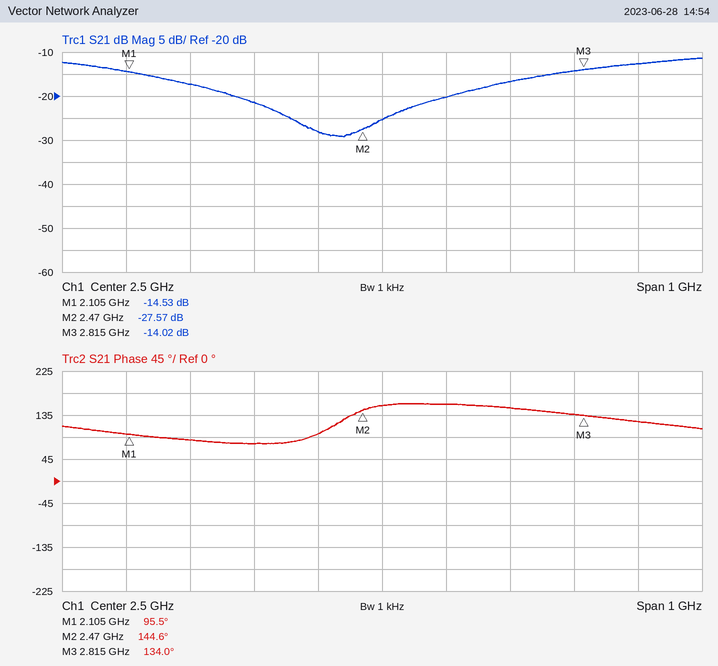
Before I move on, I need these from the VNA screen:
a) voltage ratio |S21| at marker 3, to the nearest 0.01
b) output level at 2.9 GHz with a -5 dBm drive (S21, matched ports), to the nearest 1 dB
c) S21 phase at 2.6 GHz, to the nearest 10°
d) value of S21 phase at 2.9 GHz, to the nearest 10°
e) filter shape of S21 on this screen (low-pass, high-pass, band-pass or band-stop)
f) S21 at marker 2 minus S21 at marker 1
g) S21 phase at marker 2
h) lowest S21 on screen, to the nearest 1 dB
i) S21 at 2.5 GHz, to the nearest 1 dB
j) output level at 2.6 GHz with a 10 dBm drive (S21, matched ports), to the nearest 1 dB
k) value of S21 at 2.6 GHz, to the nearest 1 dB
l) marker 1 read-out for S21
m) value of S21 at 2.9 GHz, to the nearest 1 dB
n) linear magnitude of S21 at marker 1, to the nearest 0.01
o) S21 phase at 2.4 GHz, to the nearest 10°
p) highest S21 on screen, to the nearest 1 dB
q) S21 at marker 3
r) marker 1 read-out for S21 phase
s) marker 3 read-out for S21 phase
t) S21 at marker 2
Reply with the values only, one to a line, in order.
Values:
0.20
-18 dBm
160°
120°
band-stop
-13.04 dB
144.6°
-29 dB
-25 dB
-10 dBm
-20 dB
-14.53 dB
-13 dB
0.19
100°
-11 dB
-14.02 dB
95.5°
134.0°
-27.57 dB
